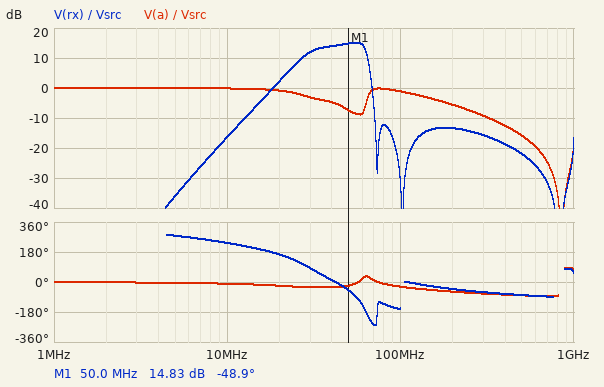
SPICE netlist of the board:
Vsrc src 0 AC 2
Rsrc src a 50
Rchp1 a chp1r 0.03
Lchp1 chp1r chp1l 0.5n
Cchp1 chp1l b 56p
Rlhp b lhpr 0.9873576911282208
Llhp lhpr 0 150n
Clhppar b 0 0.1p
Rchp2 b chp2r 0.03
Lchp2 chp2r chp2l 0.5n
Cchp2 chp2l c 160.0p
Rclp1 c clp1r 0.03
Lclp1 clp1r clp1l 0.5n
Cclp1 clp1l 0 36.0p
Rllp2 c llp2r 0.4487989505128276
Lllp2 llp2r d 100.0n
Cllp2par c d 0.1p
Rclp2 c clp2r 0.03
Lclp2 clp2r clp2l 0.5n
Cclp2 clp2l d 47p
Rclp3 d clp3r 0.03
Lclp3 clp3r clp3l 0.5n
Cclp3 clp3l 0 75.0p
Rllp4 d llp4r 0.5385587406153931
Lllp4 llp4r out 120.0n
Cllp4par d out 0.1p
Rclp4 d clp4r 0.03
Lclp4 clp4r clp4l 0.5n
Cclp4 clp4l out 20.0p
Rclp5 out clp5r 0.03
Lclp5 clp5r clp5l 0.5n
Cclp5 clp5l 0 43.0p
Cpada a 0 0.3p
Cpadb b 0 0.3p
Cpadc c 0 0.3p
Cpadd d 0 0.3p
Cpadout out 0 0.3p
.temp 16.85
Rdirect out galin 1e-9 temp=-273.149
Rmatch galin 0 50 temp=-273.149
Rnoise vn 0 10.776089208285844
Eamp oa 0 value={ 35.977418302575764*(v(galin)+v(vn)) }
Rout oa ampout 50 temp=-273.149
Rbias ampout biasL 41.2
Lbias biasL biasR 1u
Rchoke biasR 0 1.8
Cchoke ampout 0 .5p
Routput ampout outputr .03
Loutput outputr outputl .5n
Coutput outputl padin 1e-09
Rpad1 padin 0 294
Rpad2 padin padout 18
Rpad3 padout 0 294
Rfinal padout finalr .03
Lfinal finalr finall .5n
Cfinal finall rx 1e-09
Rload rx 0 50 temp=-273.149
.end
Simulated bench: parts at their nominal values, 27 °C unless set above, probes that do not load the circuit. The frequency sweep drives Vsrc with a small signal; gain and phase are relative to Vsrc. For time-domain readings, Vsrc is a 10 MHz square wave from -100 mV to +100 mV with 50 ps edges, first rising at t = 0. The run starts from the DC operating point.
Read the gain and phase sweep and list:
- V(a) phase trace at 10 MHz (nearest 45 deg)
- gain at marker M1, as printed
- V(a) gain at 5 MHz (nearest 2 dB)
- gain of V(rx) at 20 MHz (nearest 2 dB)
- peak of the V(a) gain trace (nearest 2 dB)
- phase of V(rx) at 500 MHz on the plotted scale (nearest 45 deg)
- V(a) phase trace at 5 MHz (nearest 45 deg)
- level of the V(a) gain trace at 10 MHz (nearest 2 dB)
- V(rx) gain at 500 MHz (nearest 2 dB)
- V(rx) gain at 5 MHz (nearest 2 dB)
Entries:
0 deg
14.83 dB
0 dB
2 dB
0 dB
-90 deg
0 deg
0 dB
-22 dB
-36 dB
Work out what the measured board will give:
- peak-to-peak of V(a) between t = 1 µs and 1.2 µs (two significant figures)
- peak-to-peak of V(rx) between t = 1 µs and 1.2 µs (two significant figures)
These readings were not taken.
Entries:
230 mV
650 mV
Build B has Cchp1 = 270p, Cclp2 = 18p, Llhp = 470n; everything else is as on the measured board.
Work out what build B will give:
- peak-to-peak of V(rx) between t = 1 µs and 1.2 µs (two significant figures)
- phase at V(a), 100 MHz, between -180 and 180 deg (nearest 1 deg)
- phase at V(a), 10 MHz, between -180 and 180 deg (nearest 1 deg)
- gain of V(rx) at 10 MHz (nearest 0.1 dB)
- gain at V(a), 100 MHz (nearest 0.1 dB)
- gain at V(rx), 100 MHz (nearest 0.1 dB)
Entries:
1.3 V
-30 deg
-52 deg
8.4 dB
-1.3 dB
-35.9 dB
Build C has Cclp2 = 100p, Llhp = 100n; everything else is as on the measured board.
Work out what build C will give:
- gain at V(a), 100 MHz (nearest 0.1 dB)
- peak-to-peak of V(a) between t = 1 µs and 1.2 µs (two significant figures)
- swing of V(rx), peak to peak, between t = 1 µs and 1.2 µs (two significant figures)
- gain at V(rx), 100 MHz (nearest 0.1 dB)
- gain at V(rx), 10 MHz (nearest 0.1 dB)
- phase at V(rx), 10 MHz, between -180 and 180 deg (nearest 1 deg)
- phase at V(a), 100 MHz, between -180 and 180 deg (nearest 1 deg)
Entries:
-1.3 dB
250 mV
320 mV
-26.8 dB
-20.1 dB
-128 deg
-30 deg
